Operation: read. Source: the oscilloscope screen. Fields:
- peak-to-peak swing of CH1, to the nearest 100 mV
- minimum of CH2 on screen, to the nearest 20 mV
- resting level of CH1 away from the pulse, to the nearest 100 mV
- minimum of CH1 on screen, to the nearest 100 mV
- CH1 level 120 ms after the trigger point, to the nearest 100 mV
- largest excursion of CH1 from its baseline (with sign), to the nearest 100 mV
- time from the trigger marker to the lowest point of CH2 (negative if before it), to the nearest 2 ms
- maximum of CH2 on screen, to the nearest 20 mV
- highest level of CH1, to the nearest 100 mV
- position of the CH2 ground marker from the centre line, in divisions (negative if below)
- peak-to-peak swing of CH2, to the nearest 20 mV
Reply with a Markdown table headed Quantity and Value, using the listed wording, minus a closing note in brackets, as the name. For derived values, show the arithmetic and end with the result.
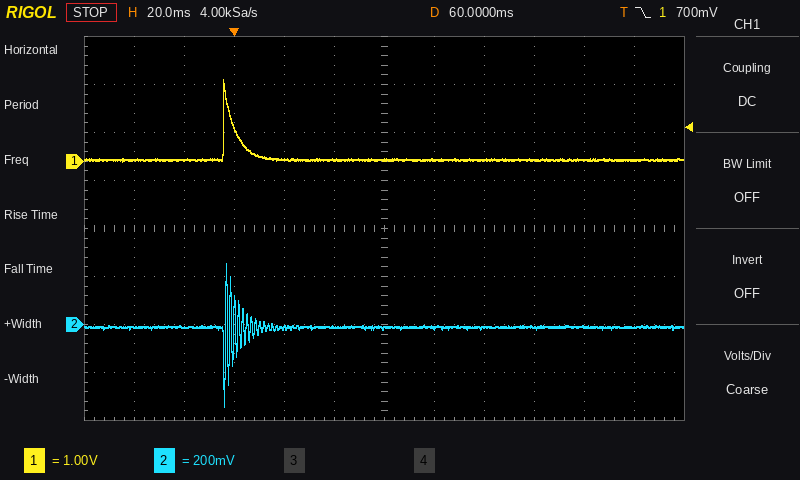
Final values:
| Quantity | Value |
|---|---|
| peak-to-peak swing of CH1, to the nearest 100 mV | 1.7 V − (0.0 V) = 1.7 V |
| minimum of CH2 on screen, to the nearest 20 mV | -340 mV |
| resting level of CH1 away from the pulse, to the nearest 100 mV | 0.0 V |
| minimum of CH1 on screen, to the nearest 100 mV | 0.0 V |
| CH1 level 120 ms after the trigger point, to the nearest 100 mV | 0.0 V |
| largest excursion of CH1 from its baseline (with sign), to the nearest 100 mV | 1.7 V − (0.0 V) = +1.7 V |
| time from the trigger marker to the lowest point of CH2 (negative if before it), to the nearest 2 ms | -4 ms |
| maximum of CH2 on screen, to the nearest 20 mV | 260 mV |
| highest level of CH1, to the nearest 100 mV | 1.7 V |
| position of the CH2 ground marker from the centre line, in divisions | -2.0 div |
| peak-to-peak swing of CH2, to the nearest 20 mV | 260 mV − (-340 mV) = 600 mV |
